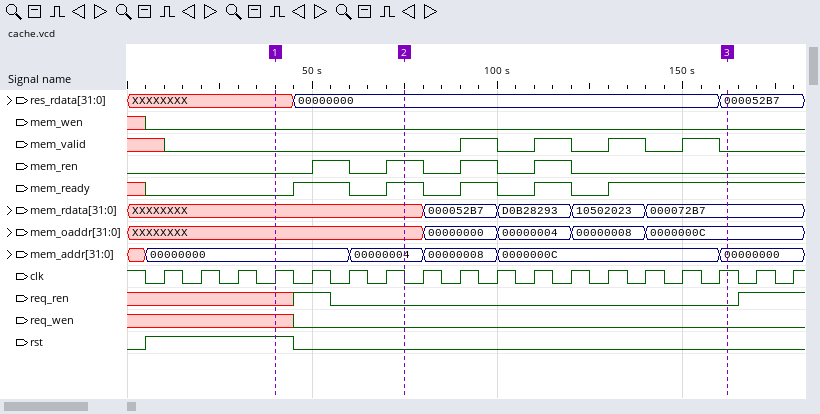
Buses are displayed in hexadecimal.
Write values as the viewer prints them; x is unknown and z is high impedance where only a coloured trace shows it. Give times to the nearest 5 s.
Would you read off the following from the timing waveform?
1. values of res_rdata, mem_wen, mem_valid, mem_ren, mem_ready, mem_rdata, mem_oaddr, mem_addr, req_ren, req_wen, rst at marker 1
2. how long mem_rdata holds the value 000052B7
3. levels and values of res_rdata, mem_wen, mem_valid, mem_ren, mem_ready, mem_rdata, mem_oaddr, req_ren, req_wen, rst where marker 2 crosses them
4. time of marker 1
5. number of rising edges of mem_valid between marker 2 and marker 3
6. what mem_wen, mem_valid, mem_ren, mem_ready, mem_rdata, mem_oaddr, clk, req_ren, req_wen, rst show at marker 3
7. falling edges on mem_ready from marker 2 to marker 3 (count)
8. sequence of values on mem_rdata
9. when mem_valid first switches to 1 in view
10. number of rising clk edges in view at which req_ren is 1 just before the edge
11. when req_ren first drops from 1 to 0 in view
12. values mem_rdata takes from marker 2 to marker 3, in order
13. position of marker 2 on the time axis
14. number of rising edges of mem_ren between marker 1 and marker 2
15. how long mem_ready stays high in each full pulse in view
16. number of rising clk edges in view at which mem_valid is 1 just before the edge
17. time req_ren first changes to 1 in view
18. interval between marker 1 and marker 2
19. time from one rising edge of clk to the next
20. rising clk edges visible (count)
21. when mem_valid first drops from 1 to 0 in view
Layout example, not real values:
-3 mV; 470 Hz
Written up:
res_rdata=XXXXXXXX, mem_wen=0, mem_valid=0, mem_ren=0, mem_ready=0, mem_rdata=XXXXXXXX, mem_oaddr=XXXXXXXX, mem_addr=00000000, req_ren=x, req_wen=x, rst=1; 20 s; res_rdata=00000000, mem_wen=0, mem_valid=0, mem_ren=1, mem_ready=1, mem_rdata=XXXXXXXX, mem_oaddr=XXXXXXXX, req_ren=0, req_wen=0, rst=0; 40 s; 4; mem_wen=0, mem_valid=0, mem_ren=0, mem_ready=1, mem_rdata=000072B7, mem_oaddr=0000000C, clk=1, req_ren=0, req_wen=0, rst=0; 3; XXXXXXXX, 000052B7, D0B28293, 10502023, 000072B7; 90 s; 3; 55 s; XXXXXXXX, 000052B7, D0B28293, 10502023, 000072B7; 75 s; 2; 15 s, 10 s, 10 s, 10 s; 4; 45 s; 35 s; 10 s; 18; 100 s
